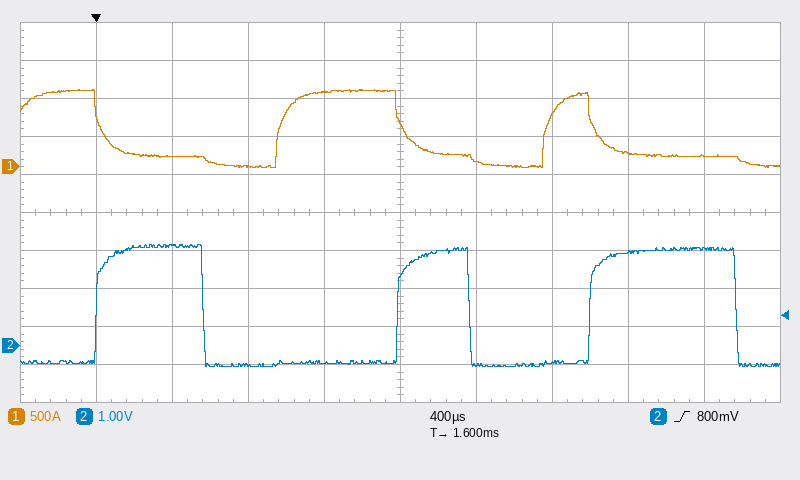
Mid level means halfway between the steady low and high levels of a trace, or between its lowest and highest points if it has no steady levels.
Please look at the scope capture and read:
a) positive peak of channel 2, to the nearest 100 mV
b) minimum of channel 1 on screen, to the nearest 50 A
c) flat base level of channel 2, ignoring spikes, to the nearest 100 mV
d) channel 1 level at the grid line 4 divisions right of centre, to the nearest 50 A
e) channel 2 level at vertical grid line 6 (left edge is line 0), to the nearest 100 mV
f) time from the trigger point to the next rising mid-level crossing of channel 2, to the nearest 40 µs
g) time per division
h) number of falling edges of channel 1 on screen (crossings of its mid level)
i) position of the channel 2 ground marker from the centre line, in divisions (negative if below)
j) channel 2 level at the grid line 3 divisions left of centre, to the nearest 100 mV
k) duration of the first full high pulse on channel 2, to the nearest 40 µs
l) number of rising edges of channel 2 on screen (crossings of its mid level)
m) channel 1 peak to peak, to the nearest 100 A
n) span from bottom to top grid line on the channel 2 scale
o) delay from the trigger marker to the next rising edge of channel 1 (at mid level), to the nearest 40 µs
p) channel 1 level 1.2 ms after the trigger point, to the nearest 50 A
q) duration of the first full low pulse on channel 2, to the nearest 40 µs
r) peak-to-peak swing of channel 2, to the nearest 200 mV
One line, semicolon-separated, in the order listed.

2.7 V; 0 A; -500 mV; 150 A; -500 mV; 1.60 ms; 400 µs; 3; -3.5 div; 2.6 V; 560 µs; 3; 1.00 kA; 10 V; 960 µs; 1.00 kA; 1.04 ms; 3.2 V
